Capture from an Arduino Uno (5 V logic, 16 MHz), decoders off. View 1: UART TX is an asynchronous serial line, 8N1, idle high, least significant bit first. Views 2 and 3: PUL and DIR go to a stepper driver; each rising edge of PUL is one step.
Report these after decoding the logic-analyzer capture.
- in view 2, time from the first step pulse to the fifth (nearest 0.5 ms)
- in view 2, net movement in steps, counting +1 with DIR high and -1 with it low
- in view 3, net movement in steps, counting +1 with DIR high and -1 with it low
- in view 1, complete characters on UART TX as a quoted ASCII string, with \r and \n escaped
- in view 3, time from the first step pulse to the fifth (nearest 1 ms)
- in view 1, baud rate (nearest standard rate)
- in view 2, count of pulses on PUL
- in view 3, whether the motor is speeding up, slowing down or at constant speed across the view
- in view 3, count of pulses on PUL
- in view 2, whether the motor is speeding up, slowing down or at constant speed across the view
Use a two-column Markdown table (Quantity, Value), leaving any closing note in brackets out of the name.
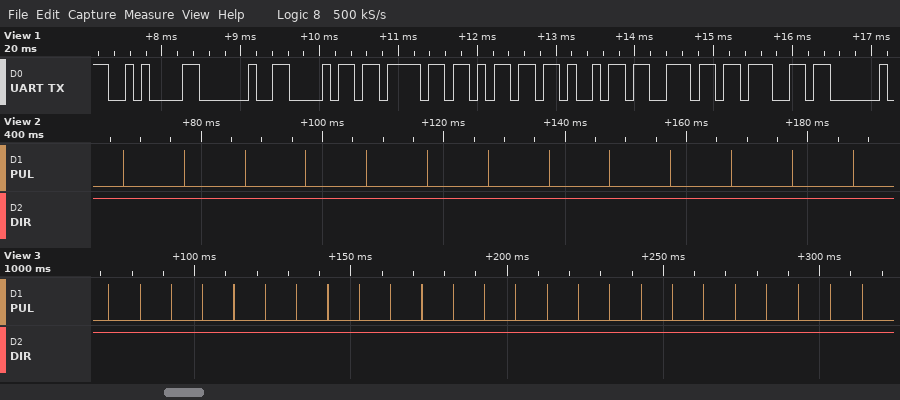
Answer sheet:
| Quantity | Value |
|---|---|
| in view 2, time from the first step pulse to the fifth | 40.0 ms |
| in view 2, net movement in steps, counting +1 with DIR high and -1 with it low | +13 |
| in view 3, net movement in steps, counting +1 with DIR high and -1 with it low | +25 |
| in view 1, complete characters on UART TX as a quoted ASCII string, with \r and \n escaped | "\n homing" |
| in view 3, time from the first step pulse to the fifth | 40 ms |
| in view 1, baud rate | 9600 baud |
| in view 2, count of pulses on PUL | 13 |
| in view 3, whether the motor is speeding up, slowing down or at constant speed across the view | constant speed |
| in view 3, count of pulses on PUL | 25 |
| in view 2, whether the motor is speeding up, slowing down or at constant speed across the view | constant speed |
